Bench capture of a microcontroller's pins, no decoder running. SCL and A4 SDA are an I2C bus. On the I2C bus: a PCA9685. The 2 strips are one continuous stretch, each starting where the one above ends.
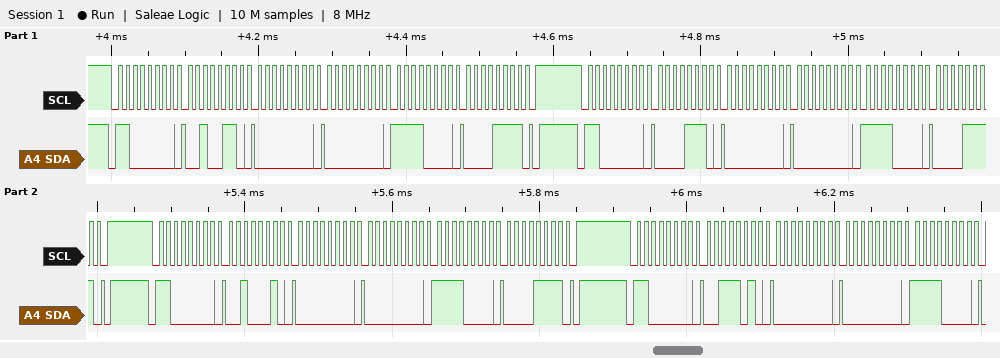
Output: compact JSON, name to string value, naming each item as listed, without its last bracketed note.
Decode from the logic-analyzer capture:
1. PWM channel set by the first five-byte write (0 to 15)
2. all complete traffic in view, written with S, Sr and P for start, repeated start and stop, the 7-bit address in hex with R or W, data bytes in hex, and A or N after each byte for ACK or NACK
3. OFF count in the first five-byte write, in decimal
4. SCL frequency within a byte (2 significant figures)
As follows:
{"PWM channel set by the first five-byte write": "8", "all complete traffic in view, written with S, Sr and P for start, repeated start and stop, the 7-bit address in hex with R or W, data bytes in hex, and A or N after each byte for ACK or NACK": "S 60W A 26 A 00 A 00 A F0 A 0F A P S 60W A 0E A 00 A 00 A F0 A 0F A P S 60W A 22 A 00 A 00 A F0 A 0F A P S 60W A 3A A 00 A 00 A F0 A", "OFF count in the first five-byte write, in decimal": "4080", "SCL frequency within a byte": "100 kHz"}
